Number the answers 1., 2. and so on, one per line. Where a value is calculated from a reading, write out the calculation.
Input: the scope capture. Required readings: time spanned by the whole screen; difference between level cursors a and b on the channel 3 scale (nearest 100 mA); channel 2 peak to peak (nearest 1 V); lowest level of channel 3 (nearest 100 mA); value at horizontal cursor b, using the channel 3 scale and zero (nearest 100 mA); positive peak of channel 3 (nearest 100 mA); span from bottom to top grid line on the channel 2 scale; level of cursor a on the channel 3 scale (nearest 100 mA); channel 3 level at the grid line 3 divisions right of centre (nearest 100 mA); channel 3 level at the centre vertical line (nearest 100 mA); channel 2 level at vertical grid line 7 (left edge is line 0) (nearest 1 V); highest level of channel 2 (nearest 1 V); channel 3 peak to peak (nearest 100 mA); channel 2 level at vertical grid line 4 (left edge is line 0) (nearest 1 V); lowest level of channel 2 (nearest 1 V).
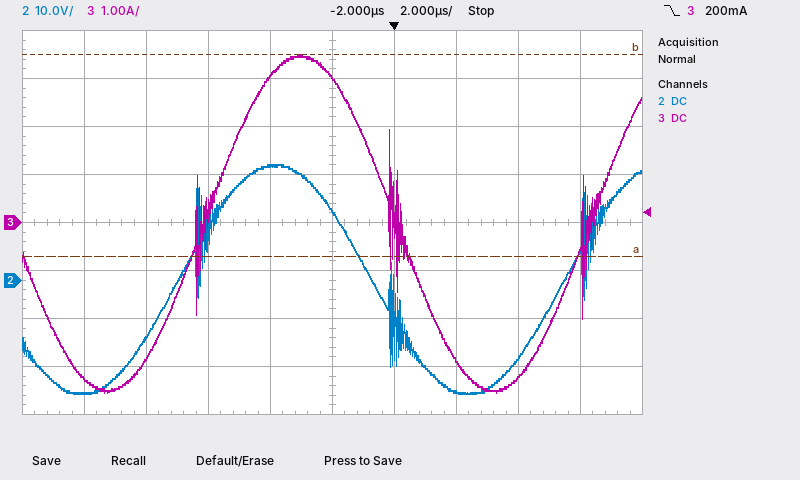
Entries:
1. 20 µs
2. 4.2 A
3. 24 V − (-24 V) = 48 V
4. -3.5 A
5. 3.5 A
6. 3.5 A
7. 80 V
8. -700 mA
9. -3.2 A
10. 3.0 A
11. -23 V
12. 24 V
13. 3.5 A − (-3.5 A) = 7.0 A
14. 24 V
15. -24 V
